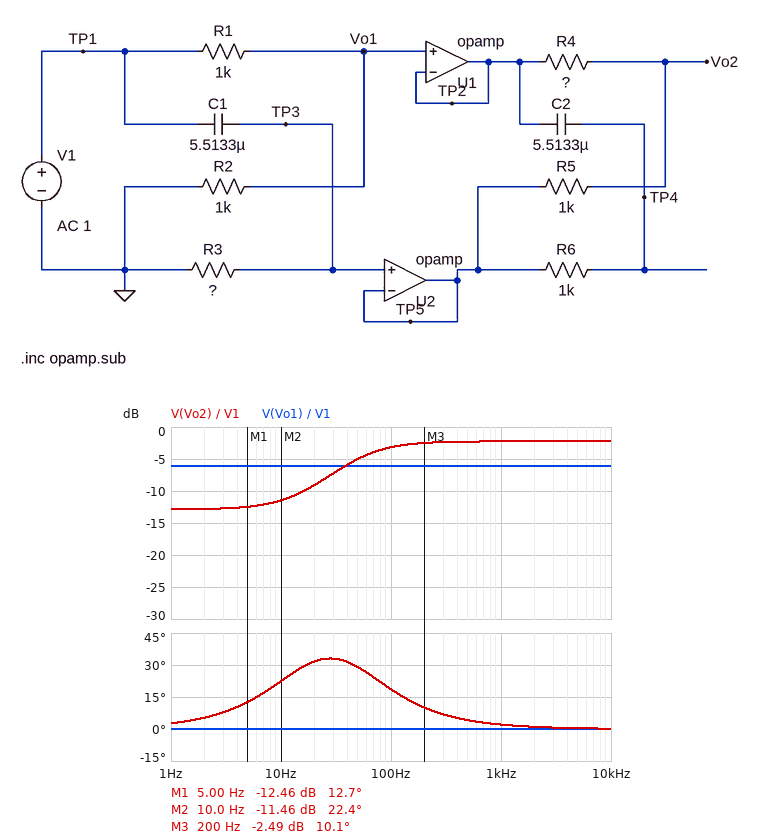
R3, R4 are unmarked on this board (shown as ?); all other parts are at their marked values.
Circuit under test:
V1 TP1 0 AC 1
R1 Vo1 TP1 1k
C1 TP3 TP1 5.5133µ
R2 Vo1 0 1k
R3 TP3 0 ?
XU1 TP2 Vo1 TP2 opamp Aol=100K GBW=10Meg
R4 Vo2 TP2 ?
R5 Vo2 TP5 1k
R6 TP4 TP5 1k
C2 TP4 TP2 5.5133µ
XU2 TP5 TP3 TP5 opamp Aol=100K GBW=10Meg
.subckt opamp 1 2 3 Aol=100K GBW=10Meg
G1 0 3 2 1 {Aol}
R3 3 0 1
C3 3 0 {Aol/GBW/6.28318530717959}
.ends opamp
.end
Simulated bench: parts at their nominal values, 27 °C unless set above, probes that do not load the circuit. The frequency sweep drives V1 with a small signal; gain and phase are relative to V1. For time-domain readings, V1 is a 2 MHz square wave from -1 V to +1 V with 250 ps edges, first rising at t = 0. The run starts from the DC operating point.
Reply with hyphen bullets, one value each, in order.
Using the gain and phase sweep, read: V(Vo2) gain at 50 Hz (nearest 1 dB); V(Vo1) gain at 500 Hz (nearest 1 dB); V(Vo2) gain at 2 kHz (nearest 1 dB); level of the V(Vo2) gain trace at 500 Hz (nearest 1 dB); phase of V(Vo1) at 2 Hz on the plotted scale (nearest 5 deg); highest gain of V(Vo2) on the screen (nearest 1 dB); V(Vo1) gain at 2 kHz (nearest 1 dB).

- -5 dB
- -6 dB
- -2 dB
- -2 dB
- 0 deg
- -2 dB
- -6 dB
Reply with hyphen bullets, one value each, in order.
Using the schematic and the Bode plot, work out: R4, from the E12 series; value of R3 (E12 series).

- 1.2 kΩ
- 560 Ω
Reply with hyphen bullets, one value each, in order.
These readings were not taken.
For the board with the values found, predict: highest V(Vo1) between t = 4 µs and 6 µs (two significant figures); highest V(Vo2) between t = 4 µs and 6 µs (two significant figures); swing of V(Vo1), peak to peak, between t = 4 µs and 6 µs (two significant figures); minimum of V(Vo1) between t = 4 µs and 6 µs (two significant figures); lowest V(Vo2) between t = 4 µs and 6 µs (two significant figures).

- 500 mV
- 1.3 V
- 1.0 V
- -500 mV
- -230 mV
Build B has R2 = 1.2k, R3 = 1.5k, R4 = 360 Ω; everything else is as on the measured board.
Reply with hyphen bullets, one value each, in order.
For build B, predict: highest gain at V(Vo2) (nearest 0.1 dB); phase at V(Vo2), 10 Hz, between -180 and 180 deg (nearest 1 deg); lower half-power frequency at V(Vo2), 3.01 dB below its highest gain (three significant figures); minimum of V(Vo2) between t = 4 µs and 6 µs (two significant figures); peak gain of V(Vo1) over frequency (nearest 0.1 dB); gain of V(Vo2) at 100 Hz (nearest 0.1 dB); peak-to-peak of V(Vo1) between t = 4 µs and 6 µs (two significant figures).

- -3.5 dB
- 13 deg
- 10.1 Hz
- -400 mV
- -5.3 dB
- -3.6 dB
- 1.1 V
